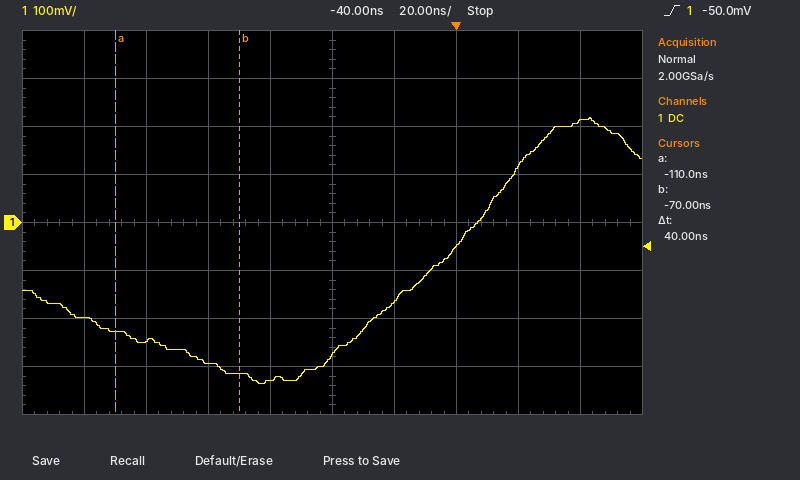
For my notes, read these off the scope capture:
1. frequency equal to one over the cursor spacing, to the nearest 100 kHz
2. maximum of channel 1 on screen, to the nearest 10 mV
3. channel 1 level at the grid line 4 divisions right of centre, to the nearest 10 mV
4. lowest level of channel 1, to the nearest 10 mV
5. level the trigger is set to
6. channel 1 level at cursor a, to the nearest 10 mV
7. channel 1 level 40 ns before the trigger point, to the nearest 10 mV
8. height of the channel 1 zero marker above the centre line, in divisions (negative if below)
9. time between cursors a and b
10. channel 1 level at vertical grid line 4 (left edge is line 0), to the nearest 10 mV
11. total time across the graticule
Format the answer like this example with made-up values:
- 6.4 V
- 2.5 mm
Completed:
- 25.0 MHz
- 220 mV
- 210 mV
- -340 mV
- -50.0 mV
- -230 mV
- -280 mV
- 0.0 div
- 40 ns
- -330 mV
- 200 ns
